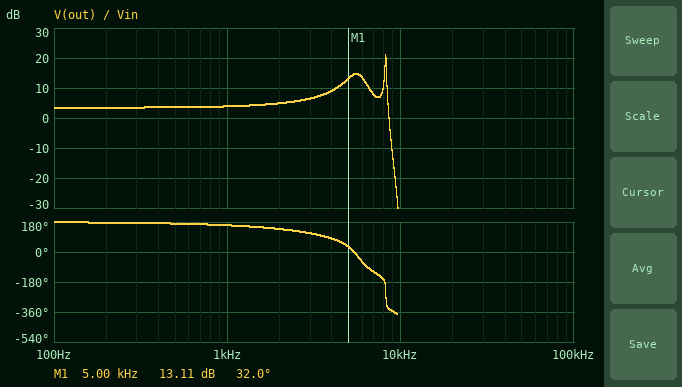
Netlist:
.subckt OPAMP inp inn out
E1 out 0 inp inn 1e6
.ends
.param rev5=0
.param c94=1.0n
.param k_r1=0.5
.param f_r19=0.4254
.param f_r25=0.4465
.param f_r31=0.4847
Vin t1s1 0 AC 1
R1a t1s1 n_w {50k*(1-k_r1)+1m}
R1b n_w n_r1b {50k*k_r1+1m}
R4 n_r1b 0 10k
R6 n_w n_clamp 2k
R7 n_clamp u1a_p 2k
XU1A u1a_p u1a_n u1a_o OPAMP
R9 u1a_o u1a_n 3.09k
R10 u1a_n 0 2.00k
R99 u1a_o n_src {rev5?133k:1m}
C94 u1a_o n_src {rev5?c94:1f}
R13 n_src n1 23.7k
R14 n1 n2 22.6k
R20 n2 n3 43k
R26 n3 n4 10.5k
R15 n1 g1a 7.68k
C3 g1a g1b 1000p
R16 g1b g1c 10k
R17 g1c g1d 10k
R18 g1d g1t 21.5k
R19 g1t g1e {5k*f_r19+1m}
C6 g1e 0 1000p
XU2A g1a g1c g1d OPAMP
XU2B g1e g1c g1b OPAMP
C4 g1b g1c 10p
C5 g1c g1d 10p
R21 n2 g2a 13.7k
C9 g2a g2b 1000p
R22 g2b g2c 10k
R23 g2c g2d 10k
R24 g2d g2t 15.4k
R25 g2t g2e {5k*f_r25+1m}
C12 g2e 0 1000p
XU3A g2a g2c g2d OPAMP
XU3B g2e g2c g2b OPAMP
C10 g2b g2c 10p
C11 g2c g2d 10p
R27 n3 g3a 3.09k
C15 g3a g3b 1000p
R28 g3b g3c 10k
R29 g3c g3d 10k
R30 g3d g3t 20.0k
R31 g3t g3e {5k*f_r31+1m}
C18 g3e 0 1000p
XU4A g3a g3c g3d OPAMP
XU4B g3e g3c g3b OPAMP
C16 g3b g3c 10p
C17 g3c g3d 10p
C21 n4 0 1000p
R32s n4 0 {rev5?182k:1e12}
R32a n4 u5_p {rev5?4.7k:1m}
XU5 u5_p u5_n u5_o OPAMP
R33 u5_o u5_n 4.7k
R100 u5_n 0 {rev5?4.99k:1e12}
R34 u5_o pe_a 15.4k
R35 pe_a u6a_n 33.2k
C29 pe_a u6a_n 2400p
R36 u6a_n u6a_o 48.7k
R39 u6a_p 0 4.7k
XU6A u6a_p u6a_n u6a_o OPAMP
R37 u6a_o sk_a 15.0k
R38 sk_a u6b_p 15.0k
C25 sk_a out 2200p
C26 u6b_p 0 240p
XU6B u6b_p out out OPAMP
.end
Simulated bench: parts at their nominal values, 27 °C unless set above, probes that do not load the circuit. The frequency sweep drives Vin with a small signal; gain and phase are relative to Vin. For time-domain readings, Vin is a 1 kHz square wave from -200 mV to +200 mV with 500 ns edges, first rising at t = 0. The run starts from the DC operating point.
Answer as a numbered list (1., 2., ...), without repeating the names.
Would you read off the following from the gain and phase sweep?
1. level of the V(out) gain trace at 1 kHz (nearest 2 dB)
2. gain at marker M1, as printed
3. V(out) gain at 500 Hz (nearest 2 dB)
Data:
1. 4 dB
2. 13.11 dB
3. 4 dB
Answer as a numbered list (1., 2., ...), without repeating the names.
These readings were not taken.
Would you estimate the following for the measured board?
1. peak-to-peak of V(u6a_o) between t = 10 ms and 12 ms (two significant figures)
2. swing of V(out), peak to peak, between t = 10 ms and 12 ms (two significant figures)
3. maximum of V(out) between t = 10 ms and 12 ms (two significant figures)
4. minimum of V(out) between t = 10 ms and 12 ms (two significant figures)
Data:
1. 1.3 V
2. 1.4 V
3. 680 mV
4. -680 mV
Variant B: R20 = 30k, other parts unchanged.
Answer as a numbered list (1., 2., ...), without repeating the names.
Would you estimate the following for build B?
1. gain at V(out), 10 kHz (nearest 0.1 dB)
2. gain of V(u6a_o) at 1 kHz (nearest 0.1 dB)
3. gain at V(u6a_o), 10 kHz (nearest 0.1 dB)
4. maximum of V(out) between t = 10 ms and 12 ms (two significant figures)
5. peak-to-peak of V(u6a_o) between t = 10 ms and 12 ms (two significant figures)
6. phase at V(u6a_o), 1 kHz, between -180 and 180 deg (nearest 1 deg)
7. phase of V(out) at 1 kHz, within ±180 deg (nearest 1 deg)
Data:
1. -38.4 dB
2. 4.1 dB
3. -41.6 dB
4. 740 mV
5. 1.4 V
6. 167 deg
7. 164 deg
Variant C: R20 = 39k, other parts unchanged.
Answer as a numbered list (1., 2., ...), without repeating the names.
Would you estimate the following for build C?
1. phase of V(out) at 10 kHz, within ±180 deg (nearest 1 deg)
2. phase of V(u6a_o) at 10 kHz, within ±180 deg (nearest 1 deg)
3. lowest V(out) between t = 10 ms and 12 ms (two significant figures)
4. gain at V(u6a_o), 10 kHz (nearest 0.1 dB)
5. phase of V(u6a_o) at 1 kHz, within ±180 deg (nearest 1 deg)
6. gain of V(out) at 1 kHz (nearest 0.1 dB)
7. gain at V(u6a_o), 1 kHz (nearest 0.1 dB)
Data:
1. -20 deg
2. 21 deg
3. -700 mV
4. -44.6 dB
5. 164 deg
6. 4.0 dB
7. 3.9 dB
